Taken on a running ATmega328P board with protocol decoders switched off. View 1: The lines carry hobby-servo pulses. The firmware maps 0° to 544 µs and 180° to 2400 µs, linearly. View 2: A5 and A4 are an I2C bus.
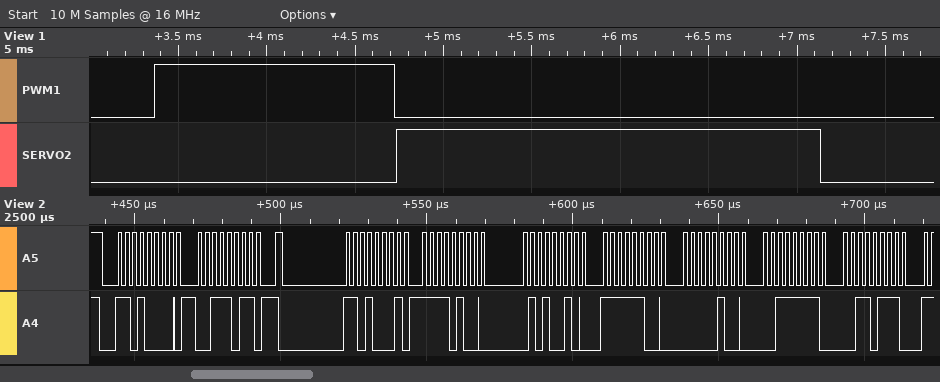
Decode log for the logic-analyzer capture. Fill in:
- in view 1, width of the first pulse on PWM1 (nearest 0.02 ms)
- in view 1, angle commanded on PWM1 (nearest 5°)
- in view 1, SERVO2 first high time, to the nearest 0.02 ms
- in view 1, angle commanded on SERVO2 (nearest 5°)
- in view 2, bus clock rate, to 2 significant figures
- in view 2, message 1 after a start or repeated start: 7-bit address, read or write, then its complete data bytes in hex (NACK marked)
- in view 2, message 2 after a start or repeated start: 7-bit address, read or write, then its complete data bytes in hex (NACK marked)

1.36 ms
80°
2.40 ms
180°
400 kHz
0x68 write: 3B
0x68 read: F4 52 FC 04 3F 37
